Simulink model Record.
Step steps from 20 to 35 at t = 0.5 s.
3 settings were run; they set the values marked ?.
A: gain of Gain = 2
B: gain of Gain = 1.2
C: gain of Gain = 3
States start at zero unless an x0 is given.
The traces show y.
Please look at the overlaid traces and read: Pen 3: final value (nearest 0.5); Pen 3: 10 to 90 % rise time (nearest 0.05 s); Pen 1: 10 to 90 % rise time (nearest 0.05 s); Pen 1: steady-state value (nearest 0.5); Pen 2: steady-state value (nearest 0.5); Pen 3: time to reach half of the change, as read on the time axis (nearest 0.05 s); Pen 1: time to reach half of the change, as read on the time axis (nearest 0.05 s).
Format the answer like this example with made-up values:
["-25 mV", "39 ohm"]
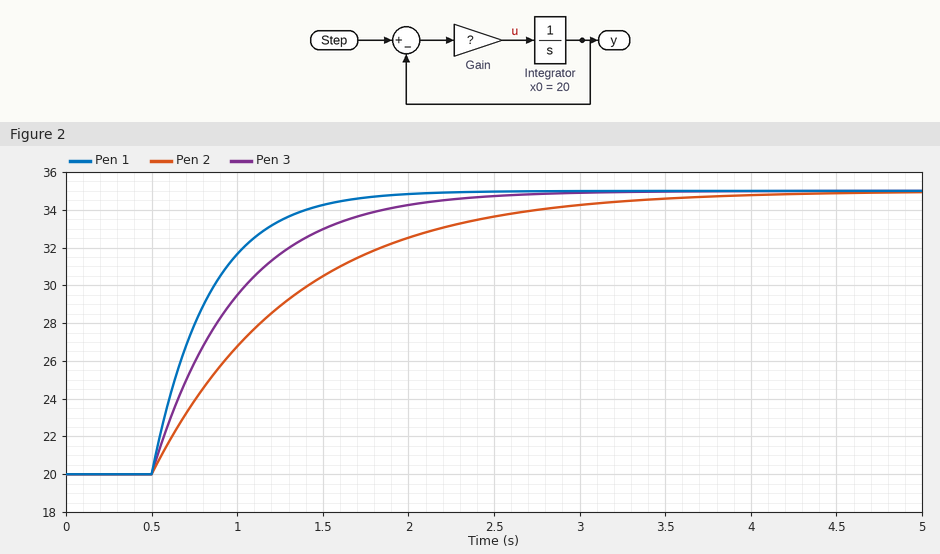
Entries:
["35.0", "1.10 s", "0.75 s", "35.0", "35.0", "0.85 s", "0.75 s"]
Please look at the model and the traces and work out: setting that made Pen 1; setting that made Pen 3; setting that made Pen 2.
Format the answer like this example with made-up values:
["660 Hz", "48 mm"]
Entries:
["C", "A", "B"]
